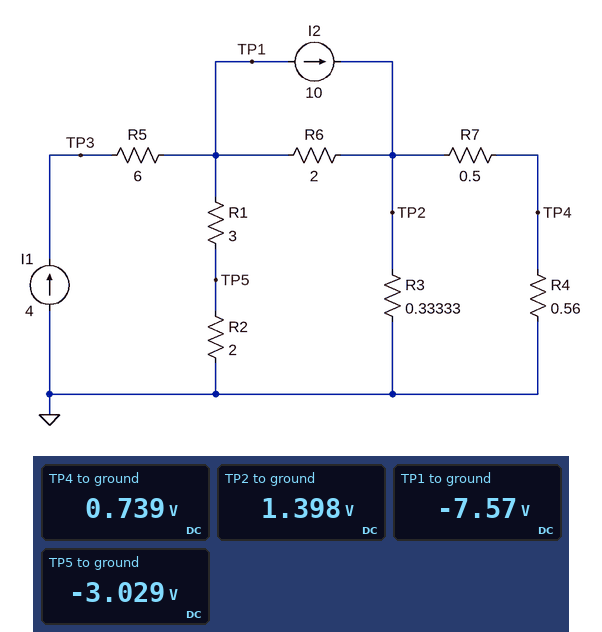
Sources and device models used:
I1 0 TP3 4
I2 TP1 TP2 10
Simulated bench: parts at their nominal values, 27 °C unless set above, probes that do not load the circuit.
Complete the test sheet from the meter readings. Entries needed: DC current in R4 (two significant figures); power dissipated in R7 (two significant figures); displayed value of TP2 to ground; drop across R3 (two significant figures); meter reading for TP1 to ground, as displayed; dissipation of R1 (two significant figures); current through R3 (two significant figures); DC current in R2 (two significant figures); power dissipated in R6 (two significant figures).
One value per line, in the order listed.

1.3 A
870 mW
1.398 V
1.4 V
-7.57 V
6.9 W
4.2 A
1.5 A
40 W
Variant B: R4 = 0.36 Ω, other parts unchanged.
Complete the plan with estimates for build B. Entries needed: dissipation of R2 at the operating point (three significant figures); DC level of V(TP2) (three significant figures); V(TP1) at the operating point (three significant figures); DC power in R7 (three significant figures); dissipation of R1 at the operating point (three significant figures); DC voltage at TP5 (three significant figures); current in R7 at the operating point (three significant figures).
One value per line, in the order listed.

4.65 W
1.33 V
-7.62 V
1.19 W
6.97 W
-3.05 V
1.54 A
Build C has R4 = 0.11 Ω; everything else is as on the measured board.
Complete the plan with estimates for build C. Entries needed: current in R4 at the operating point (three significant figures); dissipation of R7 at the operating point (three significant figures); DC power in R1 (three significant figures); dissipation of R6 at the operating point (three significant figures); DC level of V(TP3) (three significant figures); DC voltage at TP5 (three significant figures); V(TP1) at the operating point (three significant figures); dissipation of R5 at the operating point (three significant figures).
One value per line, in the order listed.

1.96 A
1.92 W
7.15 W
39.7 W
16.3 V
-3.09 V
-7.72 V
96.0 W
